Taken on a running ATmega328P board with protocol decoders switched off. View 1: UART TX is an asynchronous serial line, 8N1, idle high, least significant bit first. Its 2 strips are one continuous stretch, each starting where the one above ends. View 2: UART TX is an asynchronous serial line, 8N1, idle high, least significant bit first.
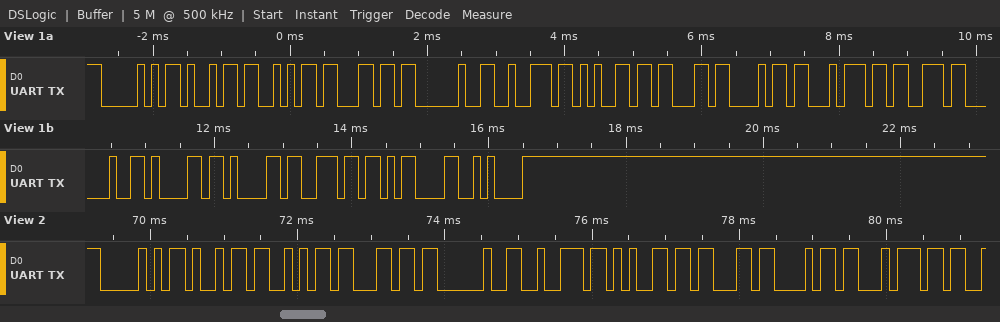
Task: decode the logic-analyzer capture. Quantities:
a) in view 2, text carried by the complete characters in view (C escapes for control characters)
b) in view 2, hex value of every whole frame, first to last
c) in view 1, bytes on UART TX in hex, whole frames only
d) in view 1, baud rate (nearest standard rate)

"Pijl recht"
50 69 6A 6C 20 72 65 63 68 74
50 69 6A 6C 20 72 65 63 68 74 73 20 61 61 6E 0D 0A
9600 baud
